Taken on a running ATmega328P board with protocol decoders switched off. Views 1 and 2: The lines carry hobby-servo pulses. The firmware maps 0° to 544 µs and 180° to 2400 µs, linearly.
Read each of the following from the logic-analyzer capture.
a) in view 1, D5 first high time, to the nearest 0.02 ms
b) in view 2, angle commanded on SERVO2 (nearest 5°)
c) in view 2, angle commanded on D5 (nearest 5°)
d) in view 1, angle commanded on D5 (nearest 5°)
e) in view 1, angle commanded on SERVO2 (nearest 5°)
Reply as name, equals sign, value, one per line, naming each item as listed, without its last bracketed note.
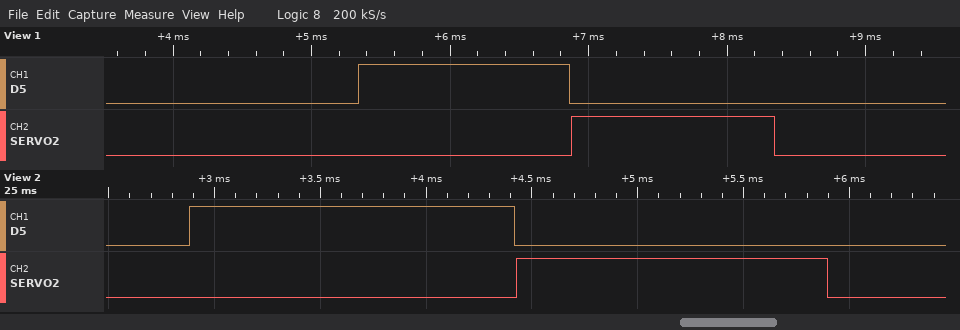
in view 1, D5 first high time, to the nearest 0.02 ms = 1.52 ms
in view 2, angle commanded on SERVO2 = 90°
in view 2, angle commanded on D5 = 95°
in view 1, angle commanded on D5 = 95°
in view 1, angle commanded on SERVO2 = 90°
